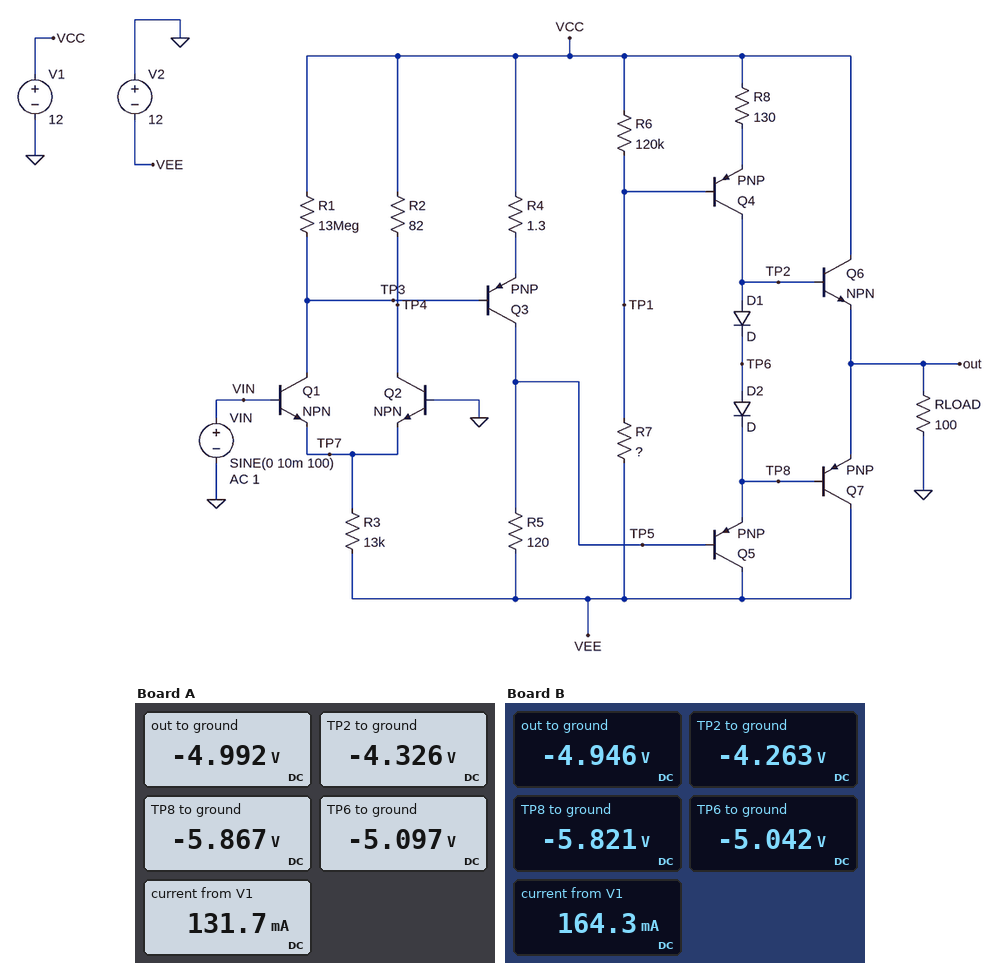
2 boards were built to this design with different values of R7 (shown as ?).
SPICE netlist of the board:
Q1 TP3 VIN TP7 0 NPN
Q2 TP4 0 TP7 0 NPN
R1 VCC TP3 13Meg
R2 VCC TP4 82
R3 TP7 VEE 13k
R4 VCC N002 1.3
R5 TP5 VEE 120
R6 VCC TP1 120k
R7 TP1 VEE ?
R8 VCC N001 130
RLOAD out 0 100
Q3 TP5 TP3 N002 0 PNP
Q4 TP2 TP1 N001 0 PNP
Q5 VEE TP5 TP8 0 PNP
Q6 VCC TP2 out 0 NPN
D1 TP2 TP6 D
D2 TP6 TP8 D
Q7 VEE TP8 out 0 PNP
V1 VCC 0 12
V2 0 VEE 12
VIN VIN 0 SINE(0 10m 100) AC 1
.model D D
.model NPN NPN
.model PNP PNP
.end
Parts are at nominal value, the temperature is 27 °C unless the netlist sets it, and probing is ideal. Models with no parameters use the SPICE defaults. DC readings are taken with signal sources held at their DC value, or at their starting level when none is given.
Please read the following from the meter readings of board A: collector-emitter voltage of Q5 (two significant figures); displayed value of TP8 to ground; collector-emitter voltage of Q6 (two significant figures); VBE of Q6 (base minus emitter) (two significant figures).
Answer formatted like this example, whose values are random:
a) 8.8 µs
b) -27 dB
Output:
a) -6.1 V
b) -5.867 V
c) 17 V
d) 670 mV
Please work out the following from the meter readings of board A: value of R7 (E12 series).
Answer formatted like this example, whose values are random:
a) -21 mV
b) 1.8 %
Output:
a) 12 kΩ
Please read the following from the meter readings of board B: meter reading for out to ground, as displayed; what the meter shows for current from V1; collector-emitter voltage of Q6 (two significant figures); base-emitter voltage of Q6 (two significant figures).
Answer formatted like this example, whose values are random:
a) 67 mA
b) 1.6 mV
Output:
a) -4.946 V
b) 164.3 mA
c) 17 V
d) 680 mV
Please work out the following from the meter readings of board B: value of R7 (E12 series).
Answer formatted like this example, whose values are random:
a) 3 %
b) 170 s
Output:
a) 5.6 kΩ
